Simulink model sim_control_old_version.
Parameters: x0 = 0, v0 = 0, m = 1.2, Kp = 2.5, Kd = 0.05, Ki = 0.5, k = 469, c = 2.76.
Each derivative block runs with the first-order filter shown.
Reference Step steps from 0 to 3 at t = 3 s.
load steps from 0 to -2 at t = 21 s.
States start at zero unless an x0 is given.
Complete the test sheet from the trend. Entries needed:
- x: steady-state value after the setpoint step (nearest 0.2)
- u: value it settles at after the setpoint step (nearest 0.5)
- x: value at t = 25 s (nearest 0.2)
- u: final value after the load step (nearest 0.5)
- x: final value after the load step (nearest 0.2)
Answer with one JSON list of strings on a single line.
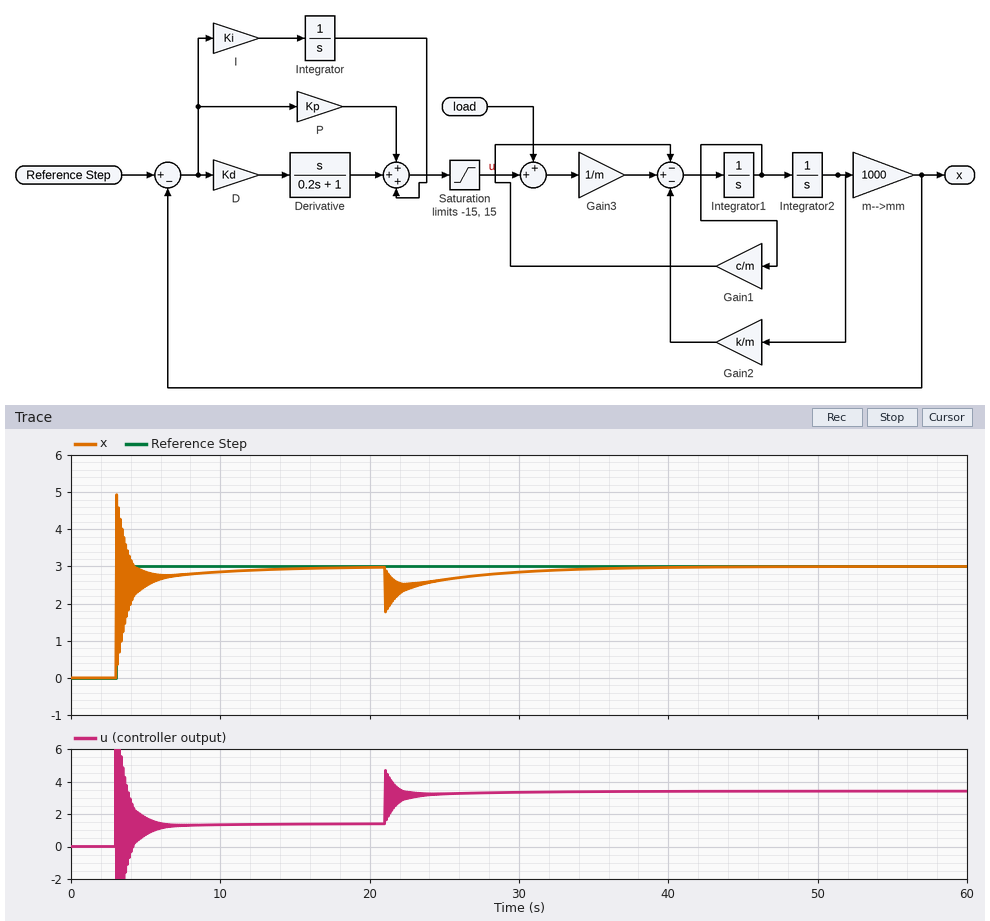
["3.0", "1.5", "2.6", "3.5", "3.0"]
